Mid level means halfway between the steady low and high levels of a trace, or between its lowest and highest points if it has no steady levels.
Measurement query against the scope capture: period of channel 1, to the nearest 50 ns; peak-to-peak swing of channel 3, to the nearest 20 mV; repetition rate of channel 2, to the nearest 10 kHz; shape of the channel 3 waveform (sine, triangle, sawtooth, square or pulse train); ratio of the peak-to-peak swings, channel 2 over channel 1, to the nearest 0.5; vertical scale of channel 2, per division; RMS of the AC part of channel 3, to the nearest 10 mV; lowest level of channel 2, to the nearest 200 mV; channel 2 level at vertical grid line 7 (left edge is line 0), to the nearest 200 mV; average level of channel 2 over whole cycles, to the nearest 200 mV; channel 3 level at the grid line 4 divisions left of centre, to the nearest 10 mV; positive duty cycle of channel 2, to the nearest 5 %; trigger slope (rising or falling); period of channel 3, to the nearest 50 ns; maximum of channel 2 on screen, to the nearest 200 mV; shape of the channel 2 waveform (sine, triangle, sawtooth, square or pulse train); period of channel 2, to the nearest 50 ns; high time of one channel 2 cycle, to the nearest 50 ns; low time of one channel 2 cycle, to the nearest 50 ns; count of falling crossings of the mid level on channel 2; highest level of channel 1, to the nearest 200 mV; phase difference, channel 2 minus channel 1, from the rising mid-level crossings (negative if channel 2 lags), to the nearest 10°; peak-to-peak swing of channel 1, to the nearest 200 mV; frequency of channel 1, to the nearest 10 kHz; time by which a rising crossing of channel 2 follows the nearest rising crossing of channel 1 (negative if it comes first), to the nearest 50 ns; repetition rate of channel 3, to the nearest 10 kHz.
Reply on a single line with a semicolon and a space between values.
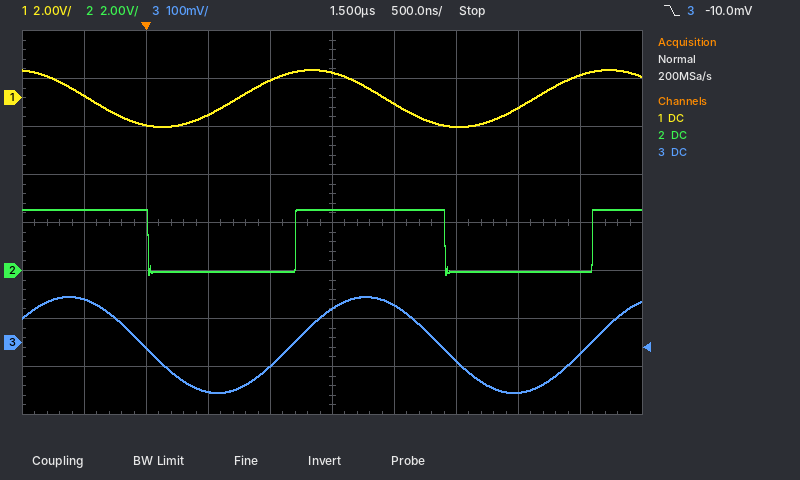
2.40 µs; 200 mV; 420 kHz; sine; 1.0; 2 V; 70 mV; -200 mV; 0.0 V; 1.2 V; 90 mV; 50 %; falling; 2.40 µs; 2.6 V; square; 2.40 µs; 1.20 µs; 1.20 µs; 2; 1.2 V; -70°; 2.4 V; 420 kHz; +450 ns; 420 kHz
